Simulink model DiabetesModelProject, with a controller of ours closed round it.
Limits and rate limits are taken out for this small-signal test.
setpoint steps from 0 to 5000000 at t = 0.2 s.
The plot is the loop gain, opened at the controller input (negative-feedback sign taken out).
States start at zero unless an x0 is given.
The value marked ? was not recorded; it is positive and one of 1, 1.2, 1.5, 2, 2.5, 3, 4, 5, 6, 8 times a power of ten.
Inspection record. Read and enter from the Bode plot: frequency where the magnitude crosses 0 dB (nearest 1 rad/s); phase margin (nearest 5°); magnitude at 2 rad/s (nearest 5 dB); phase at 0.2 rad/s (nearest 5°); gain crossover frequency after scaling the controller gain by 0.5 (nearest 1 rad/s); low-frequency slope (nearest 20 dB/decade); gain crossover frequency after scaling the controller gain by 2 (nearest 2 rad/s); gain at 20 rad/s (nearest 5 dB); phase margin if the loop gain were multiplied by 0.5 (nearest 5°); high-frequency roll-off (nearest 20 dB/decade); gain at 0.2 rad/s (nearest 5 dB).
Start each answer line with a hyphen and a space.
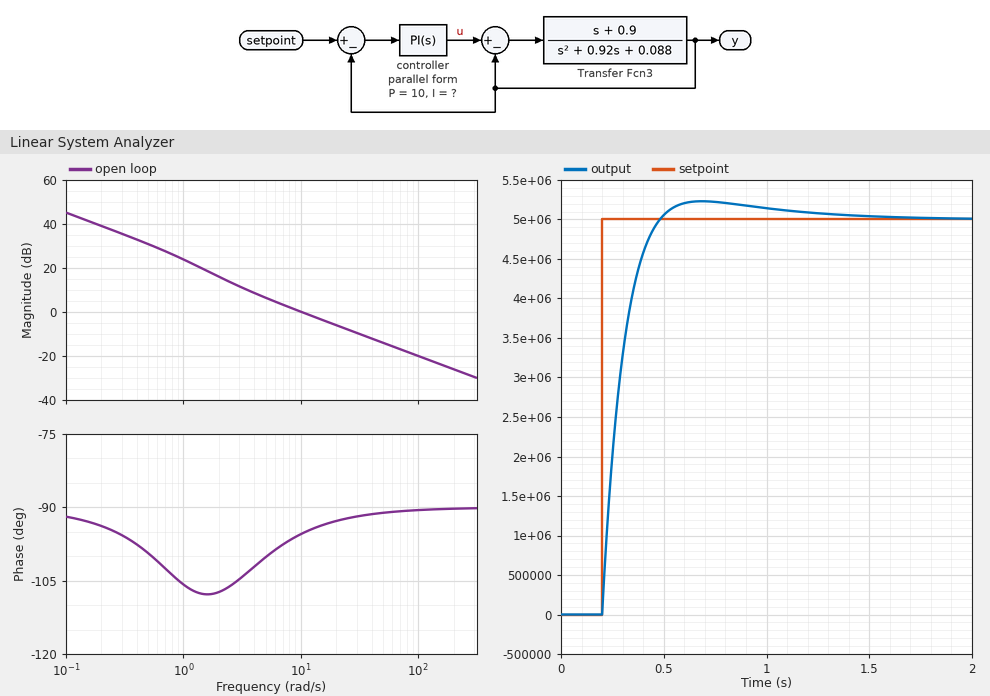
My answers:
- 10 rad/s
- 85°
- 15 dB
- -95°
- 5 rad/s
- -20 dB/decade
- 20 rad/s
- -5 dB
- 80°
- -20 dB/decade
- 40 dB
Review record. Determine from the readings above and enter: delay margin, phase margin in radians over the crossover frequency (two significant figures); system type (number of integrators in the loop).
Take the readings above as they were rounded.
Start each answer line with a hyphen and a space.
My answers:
- 0.15 s
- 1
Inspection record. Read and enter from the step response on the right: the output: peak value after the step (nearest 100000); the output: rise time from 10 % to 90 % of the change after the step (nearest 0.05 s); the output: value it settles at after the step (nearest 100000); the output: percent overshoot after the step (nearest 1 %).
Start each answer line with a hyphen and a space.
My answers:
- 5200000
- 0.20 s
- 5000000
- 5 %
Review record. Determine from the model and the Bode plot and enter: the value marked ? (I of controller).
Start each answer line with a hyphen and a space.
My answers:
- 20
